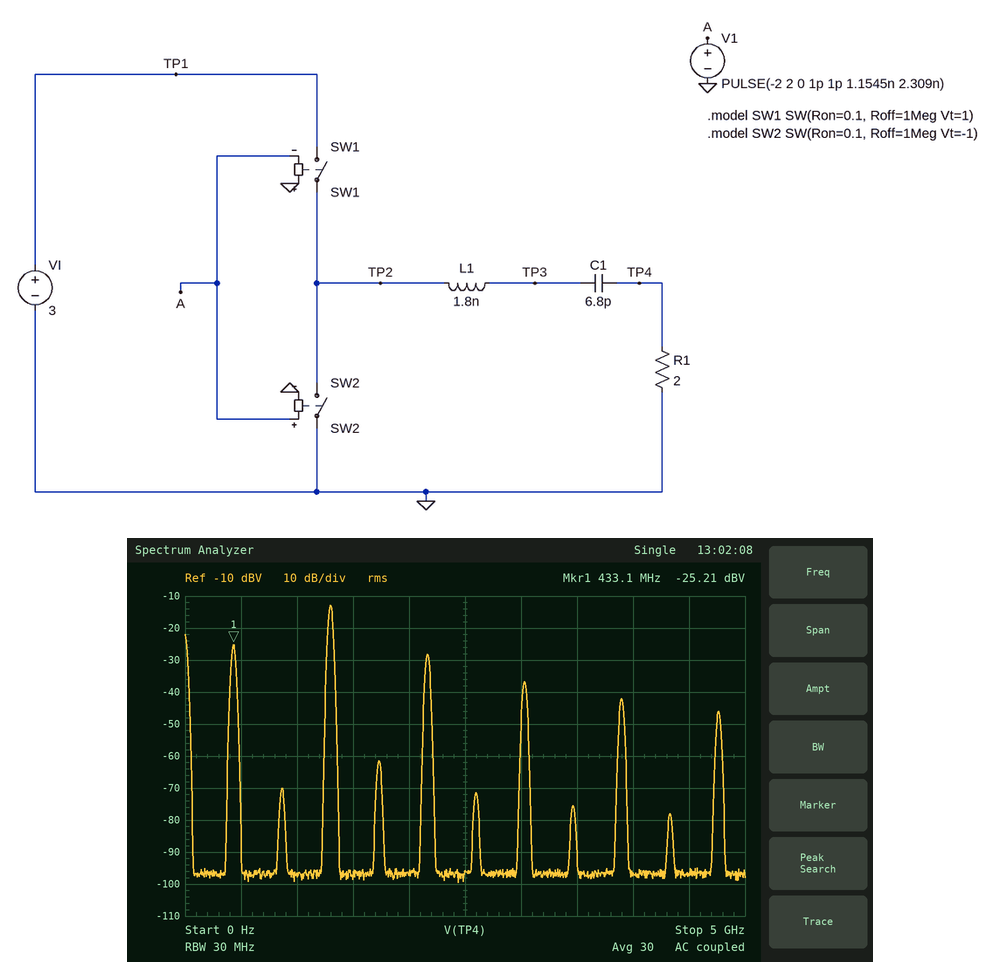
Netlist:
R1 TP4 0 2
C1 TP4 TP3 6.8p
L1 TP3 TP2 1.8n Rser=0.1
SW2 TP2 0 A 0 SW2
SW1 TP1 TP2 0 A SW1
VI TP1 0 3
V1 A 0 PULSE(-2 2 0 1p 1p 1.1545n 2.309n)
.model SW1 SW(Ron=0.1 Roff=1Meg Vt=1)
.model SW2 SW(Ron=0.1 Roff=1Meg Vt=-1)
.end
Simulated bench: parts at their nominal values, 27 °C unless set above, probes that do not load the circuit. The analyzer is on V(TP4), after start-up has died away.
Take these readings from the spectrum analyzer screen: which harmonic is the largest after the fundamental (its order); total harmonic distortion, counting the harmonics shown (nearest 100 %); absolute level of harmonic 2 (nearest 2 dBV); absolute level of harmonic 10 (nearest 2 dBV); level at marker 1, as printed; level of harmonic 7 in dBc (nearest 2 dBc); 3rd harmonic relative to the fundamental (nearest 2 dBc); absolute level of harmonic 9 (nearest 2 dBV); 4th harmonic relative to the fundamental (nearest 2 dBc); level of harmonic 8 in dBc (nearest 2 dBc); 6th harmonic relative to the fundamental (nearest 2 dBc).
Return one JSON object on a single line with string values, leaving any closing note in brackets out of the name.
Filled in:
{"which harmonic is the largest after the fundamental": "3", "total harmonic distortion, counting the harmonics shown": "400 %", "absolute level of harmonic 2": "-70 dBV", "absolute level of harmonic 10": "-78 dBV", "level at marker 1, as printed": "-25.21 dBV", "level of harmonic 7 in dBc": "-12 dBc", "3rd harmonic relative to the fundamental": "12 dBc", "absolute level of harmonic 9": "-42 dBV", "4th harmonic relative to the fundamental": "-36 dBc", "level of harmonic 8 in dBc": "-50 dBc", "6th harmonic relative to the fundamental": "-46 dBc"}
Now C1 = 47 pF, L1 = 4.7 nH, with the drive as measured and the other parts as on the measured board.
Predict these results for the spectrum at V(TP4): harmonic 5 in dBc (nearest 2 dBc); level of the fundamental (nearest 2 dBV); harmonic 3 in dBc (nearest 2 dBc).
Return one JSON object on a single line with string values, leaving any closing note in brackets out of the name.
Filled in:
{"harmonic 5 in dBc": "-36 dBc", "level of the fundamental": "-6 dBV", "harmonic 3 in dBc": "-26 dBc"}
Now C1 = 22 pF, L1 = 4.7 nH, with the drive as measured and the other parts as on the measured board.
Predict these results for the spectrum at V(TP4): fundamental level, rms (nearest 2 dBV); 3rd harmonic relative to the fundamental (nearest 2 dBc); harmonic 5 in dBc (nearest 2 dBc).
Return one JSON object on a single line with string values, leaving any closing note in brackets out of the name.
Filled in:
{"fundamental level, rms": "-4 dBV", "3rd harmonic relative to the fundamental": "-26 dBc", "harmonic 5 in dBc": "-36 dBc"}
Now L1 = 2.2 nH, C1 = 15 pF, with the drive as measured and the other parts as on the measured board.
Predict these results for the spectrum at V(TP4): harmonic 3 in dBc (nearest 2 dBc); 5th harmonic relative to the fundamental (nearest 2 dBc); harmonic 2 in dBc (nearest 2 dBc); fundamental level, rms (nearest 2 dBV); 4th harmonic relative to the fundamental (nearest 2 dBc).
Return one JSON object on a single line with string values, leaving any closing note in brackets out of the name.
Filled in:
{"harmonic 3 in dBc": "-4 dBc", "5th harmonic relative to the fundamental": "-16 dBc", "harmonic 2 in dBc": "-36 dBc", "fundamental level, rms": "-16 dBV", "4th harmonic relative to the fundamental": "-54 dBc"}
